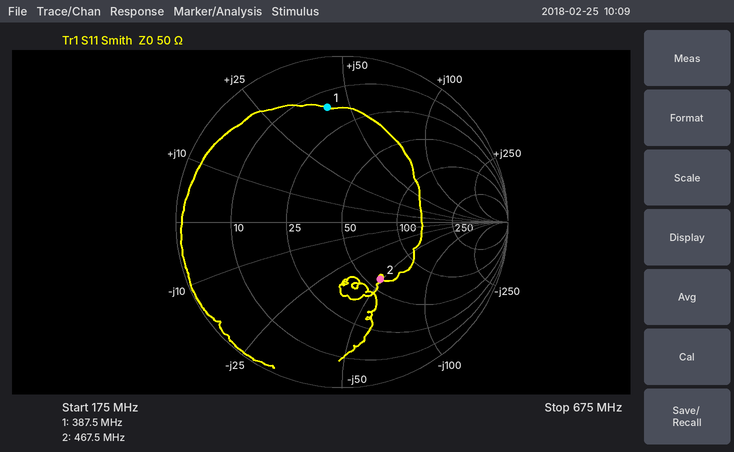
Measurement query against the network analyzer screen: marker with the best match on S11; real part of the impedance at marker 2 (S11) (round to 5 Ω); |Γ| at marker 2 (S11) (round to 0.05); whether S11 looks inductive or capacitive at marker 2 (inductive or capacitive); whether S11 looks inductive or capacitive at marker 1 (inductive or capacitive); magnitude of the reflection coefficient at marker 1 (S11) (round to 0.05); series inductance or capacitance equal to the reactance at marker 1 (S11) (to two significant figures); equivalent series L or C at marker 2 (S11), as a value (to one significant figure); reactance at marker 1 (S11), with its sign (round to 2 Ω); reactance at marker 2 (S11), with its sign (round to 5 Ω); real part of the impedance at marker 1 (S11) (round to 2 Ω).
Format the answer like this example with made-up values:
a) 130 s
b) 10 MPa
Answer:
a) marker 2
b) 60 Ω
c) 0.40
d) capacitive
e) inductive
f) 0.70
g) 17 nH
h) 7 pF
i) +42 Ω
j) -50 Ω
k) 16 Ω
